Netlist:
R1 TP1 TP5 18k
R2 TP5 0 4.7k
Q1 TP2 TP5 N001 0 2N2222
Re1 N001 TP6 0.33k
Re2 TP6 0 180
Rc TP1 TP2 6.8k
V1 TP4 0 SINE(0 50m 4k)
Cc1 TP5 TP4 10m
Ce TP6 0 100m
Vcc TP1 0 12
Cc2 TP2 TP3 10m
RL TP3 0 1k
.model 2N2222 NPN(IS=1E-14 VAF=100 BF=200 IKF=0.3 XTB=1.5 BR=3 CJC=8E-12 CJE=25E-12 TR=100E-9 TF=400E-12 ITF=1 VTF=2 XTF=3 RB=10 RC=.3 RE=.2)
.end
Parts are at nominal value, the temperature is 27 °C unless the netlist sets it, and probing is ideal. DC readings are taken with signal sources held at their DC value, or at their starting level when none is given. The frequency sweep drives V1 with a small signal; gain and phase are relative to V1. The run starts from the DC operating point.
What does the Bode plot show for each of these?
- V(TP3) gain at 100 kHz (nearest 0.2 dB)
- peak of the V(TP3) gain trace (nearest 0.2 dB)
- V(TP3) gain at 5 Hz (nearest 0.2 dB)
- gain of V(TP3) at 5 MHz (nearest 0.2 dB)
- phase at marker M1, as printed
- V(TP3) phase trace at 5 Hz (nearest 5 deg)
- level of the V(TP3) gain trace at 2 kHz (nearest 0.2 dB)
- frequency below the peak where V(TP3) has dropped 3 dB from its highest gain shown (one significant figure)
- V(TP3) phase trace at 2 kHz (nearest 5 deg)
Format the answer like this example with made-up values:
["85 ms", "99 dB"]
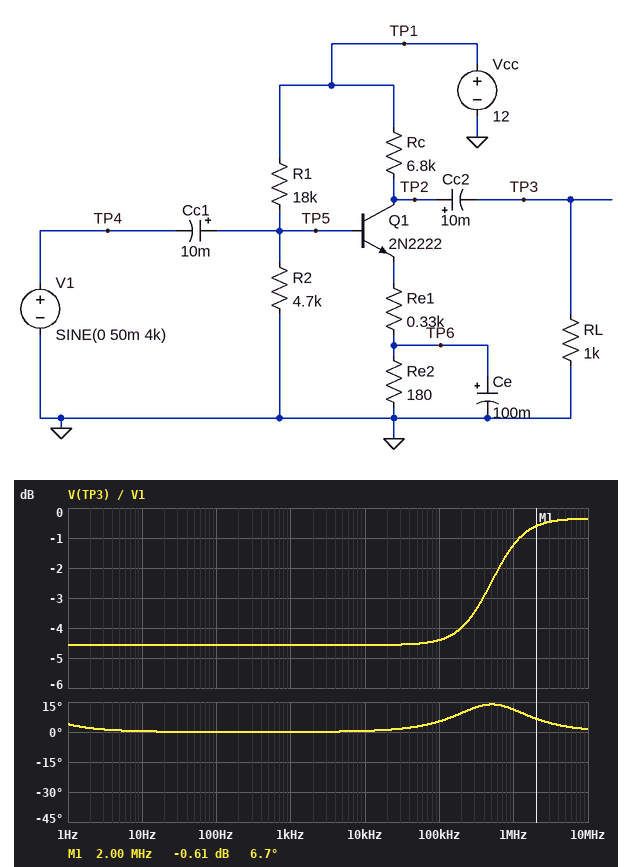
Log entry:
["-4.4 dB", "-0.4 dB", "-4.6 dB", "-0.4 dB", "6.7 deg", "0 deg", "-4.6 dB", "300 kHz", "0 deg"]
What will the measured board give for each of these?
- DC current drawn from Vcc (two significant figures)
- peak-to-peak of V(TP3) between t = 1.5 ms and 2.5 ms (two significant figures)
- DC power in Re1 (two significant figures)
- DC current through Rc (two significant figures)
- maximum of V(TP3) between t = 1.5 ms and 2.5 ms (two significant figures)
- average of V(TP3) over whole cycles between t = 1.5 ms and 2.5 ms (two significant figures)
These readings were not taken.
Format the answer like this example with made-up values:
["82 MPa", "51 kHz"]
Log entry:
["2.2 mA", "53 mV", "1.1 mW", "1.6 mA", "34 mV", "3.4 mV"]
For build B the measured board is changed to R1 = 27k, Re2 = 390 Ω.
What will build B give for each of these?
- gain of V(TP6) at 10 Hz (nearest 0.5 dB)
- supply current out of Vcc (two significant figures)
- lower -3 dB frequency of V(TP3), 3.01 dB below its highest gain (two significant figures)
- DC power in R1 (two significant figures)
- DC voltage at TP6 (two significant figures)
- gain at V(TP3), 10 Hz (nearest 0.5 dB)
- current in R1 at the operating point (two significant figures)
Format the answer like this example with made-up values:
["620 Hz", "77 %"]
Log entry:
["-67.0 dB", "1.9 mA", "9.3 mHz", "3.9 mW", "590 mV", "8.0 dB", "380 µA"]
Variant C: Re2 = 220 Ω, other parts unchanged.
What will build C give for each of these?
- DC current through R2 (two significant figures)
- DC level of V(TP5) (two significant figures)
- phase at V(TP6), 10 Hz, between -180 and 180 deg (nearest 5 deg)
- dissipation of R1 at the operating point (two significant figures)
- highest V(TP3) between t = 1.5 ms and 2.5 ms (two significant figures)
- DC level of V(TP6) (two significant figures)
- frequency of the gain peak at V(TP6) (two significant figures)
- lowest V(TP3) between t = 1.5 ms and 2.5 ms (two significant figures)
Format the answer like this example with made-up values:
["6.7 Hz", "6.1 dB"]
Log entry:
["360 µA", "1.7 V", "-90 deg", "5.9 mW", "33 mV", "400 mV", "19 mHz", "-17 mV"]
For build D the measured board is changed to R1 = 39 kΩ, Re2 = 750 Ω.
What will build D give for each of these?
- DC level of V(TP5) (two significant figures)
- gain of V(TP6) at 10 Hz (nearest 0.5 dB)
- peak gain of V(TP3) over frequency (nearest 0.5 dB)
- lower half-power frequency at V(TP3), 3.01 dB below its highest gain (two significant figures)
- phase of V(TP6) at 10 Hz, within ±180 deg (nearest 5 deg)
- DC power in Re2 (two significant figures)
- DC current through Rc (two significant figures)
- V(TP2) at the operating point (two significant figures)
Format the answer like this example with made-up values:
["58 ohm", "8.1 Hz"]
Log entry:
["1.3 V", "-67.5 dB", "7.5 dB", "8.2 mHz", "-90 deg", "260 µW", "590 µA", "8.0 V"]
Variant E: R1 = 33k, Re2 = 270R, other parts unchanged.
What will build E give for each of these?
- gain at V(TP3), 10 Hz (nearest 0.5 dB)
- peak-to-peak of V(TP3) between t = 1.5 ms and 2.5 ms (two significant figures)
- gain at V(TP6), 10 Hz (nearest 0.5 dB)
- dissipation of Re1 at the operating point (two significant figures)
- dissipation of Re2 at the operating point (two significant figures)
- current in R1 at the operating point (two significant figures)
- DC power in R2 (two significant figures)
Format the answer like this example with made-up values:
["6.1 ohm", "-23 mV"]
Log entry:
["8.0 dB", "250 mV", "-67.0 dB", "600 µW", "490 µW", "320 µA", "460 µW"]
